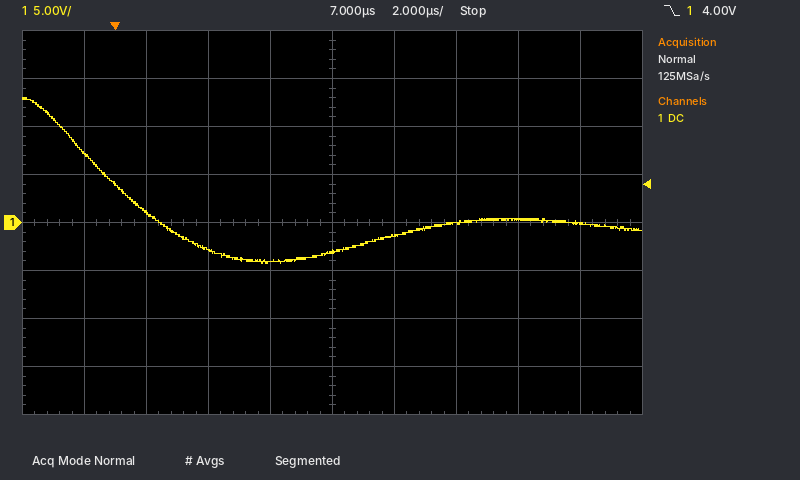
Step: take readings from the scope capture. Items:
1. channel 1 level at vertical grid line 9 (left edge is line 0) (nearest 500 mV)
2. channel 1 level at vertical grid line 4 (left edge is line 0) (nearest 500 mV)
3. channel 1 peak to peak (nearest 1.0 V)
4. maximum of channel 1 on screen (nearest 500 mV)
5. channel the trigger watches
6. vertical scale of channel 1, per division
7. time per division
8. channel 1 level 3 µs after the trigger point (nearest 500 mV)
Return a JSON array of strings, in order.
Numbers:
["0.0 V", "-4.0 V", "17.0 V", "13.0 V", "channel 1", "5 V", "2 µs", "-3.0 V"]
